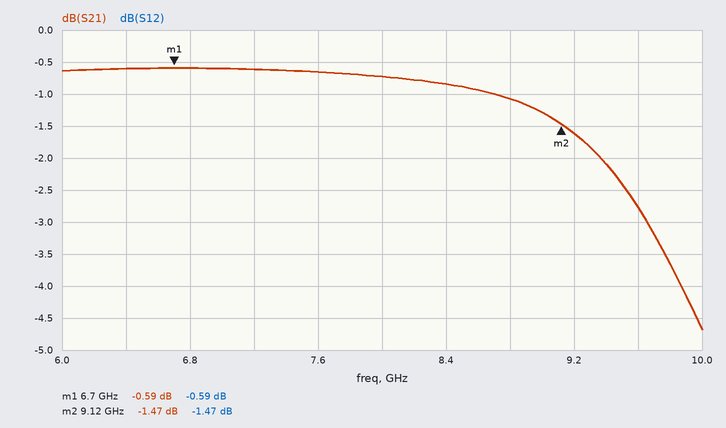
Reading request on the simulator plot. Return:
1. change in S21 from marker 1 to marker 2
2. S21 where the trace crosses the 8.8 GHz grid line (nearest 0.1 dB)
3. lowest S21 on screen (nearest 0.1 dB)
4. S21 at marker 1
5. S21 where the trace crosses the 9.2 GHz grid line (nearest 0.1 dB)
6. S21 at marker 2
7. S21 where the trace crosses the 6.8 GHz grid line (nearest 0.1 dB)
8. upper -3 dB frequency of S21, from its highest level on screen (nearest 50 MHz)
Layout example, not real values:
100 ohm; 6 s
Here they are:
-0.88 dB; -1.1 dB; -4.7 dB; -0.59 dB; -1.6 dB; -1.47 dB; -0.6 dB; 9.80 GHz
